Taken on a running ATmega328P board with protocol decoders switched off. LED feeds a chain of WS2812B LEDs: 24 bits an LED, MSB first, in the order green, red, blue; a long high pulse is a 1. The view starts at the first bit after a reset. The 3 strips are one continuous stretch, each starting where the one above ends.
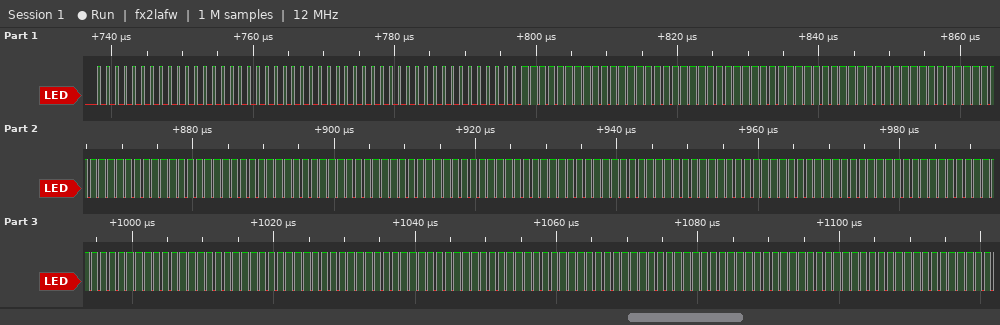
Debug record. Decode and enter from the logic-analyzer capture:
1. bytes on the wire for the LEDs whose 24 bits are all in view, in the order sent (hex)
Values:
00 00 00 00 00 00 FF FF FF FF FF FF FF FF FF FF FF FF FF FF FF FF FF FF FF FF FF FF FF FF FF FF FF FF FF FF
